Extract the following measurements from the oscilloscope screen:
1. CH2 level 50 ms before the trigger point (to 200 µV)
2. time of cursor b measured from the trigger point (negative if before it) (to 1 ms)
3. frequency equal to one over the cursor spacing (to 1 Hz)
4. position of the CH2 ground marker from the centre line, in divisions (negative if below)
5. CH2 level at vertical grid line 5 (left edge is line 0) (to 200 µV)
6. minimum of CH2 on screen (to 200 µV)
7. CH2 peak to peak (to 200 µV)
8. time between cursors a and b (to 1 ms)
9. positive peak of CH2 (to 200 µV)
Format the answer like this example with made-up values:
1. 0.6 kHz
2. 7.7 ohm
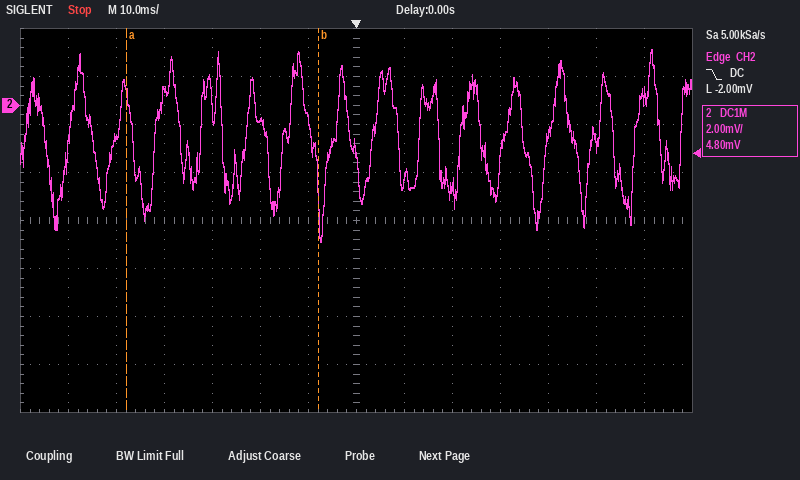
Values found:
1. -1.4 mV
2. -8 ms
3. 25 Hz
4. +2.4 div
5. -600 µV
6. -5.6 mV
7. 8.0 mV
8. 40 ms
9. 2.4 mV
